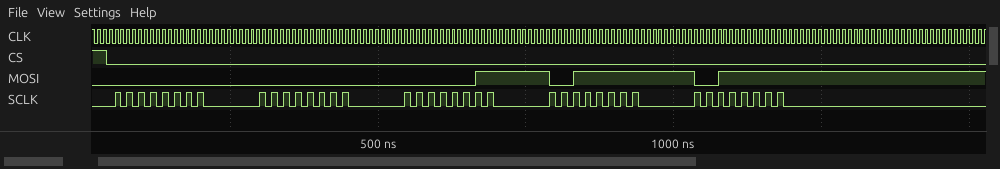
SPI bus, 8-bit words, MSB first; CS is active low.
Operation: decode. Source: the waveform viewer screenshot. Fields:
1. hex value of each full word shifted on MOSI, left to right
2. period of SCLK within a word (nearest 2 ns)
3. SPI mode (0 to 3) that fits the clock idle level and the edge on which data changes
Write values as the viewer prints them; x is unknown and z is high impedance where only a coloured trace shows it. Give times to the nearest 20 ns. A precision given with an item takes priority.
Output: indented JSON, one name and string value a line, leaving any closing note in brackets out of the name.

{
  "hex value of each full word shifted on MOSI, left to right": "00, 00, 03, 3F, 3F",
  "period of SCLK within a word": "20 ns",
  "SPI mode (0 to 3) that fits the clock idle level and the edge on which data changes": "1"
}
